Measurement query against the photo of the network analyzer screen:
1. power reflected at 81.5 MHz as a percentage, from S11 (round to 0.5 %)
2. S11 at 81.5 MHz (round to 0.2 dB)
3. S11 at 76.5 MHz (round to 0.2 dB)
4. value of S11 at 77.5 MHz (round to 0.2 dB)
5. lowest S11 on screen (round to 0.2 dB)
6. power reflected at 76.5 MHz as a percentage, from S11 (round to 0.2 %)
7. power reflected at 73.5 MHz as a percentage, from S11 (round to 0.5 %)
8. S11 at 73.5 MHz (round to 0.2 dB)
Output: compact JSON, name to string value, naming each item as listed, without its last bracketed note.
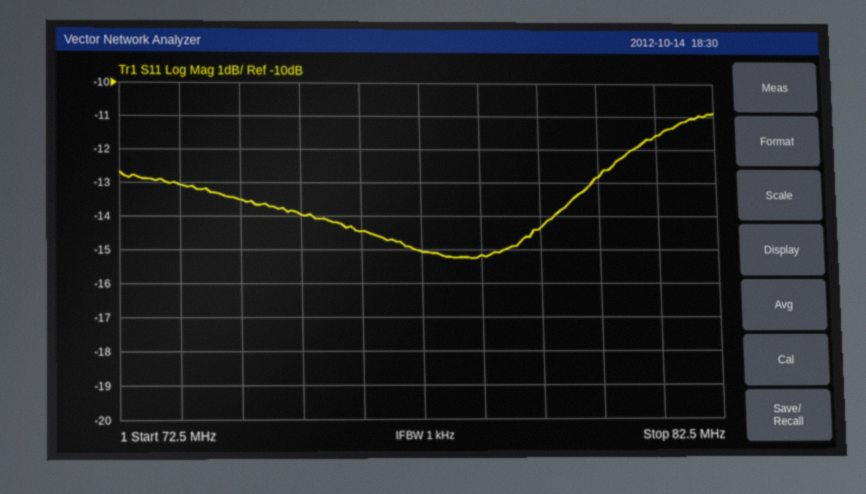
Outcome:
{"power reflected at 81.5 MHz as a percentage, from S11": "7.0 %", "S11 at 81.5 MHz": "-11.6 dB", "S11 at 76.5 MHz": "-14.4 dB", "value of S11 at 77.5 MHz": "-15.0 dB", "lowest S11 on screen": "-15.2 dB", "power reflected at 76.5 MHz as a percentage, from S11": "3.6 %", "power reflected at 73.5 MHz as a percentage, from S11": "5.0 %", "S11 at 73.5 MHz": "-13.0 dB"}
